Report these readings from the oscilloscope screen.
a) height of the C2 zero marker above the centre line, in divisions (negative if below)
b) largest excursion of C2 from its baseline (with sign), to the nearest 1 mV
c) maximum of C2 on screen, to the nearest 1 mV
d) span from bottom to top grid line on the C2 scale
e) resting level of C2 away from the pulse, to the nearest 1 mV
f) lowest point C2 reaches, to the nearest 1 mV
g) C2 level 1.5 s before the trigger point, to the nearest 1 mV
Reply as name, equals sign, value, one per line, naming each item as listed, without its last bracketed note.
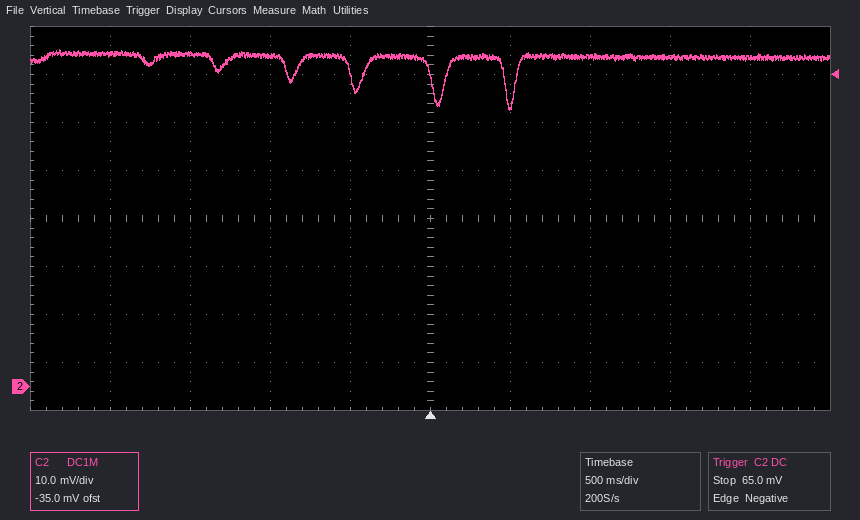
height of the C2 zero marker above the centre line, in divisions = -3.5 div
largest excursion of C2 from its baseline (with sign), to the nearest 1 mV = -11 mV
maximum of C2 on screen, to the nearest 1 mV = 70 mV
span from bottom to top grid line on the C2 scale = 80 mV
resting level of C2 away from the pulse, to the nearest 1 mV = 69 mV
lowest point C2 reaches, to the nearest 1 mV = 58 mV
C2 level 1.5 s before the trigger point, to the nearest 1 mV = 69 mV
